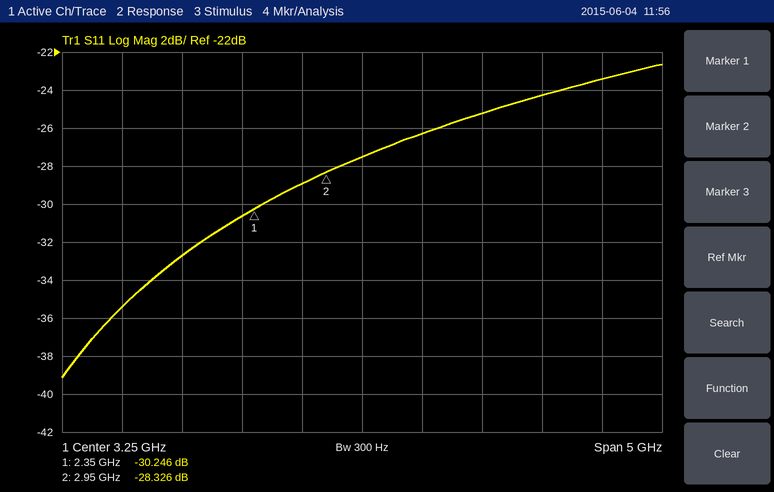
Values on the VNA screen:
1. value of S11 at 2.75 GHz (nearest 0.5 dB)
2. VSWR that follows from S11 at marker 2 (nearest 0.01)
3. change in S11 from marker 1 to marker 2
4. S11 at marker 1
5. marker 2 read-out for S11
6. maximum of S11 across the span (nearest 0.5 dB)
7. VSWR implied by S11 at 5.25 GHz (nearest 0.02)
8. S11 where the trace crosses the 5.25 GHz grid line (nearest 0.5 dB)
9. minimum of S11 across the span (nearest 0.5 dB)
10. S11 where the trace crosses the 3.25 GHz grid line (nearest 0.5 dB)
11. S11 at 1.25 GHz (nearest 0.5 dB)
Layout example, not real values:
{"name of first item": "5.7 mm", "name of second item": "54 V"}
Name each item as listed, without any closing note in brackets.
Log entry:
{"value of S11 at 2.75 GHz": "-29.0 dB", "VSWR that follows from S11 at marker 2": "1.08", "change in S11 from marker 1 to marker 2": "1.920 dB", "S11 at marker 1": "-30.246 dB", "marker 2 read-out for S11": "-28.326 dB", "maximum of S11 across the span": "-22.5 dB", "VSWR implied by S11 at 5.25 GHz": "1.14", "S11 where the trace crosses the 5.25 GHz grid line": "-23.5 dB", "minimum of S11 across the span": "-39.0 dB", "S11 where the trace crosses the 3.25 GHz grid line": "-27.5 dB", "S11 at 1.25 GHz": "-35.5 dB"}
